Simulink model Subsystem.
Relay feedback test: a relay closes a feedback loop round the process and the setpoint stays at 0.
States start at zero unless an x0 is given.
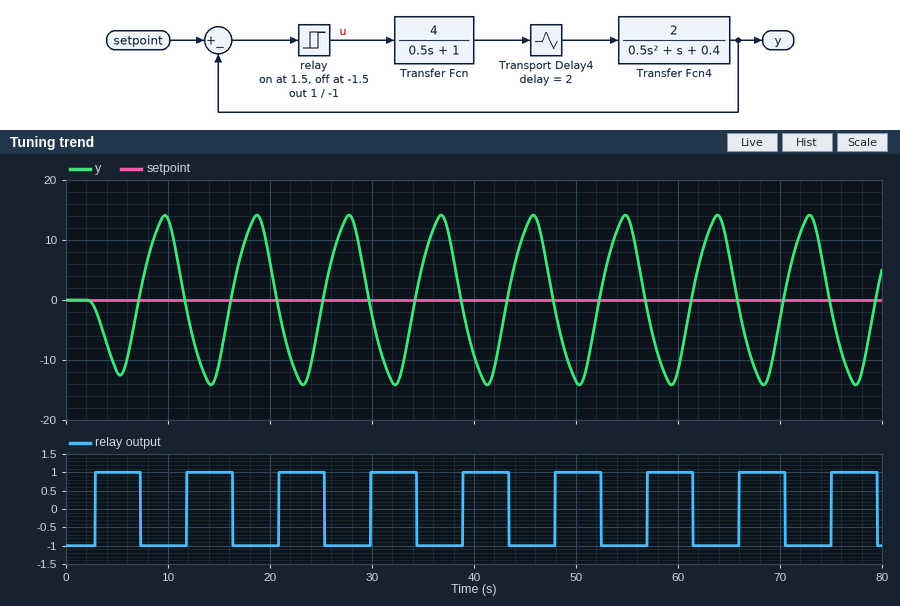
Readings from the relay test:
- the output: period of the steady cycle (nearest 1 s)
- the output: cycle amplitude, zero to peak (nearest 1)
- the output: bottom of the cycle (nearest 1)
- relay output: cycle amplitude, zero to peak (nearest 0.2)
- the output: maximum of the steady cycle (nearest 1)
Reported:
9 s
14
-14
1.0
14
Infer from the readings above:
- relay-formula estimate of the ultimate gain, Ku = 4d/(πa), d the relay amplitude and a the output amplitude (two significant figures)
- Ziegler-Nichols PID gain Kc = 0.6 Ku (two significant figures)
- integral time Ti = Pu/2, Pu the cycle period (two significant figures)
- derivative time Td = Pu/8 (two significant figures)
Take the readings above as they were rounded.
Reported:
0.091
0.055
4.5 s
1.1 s
